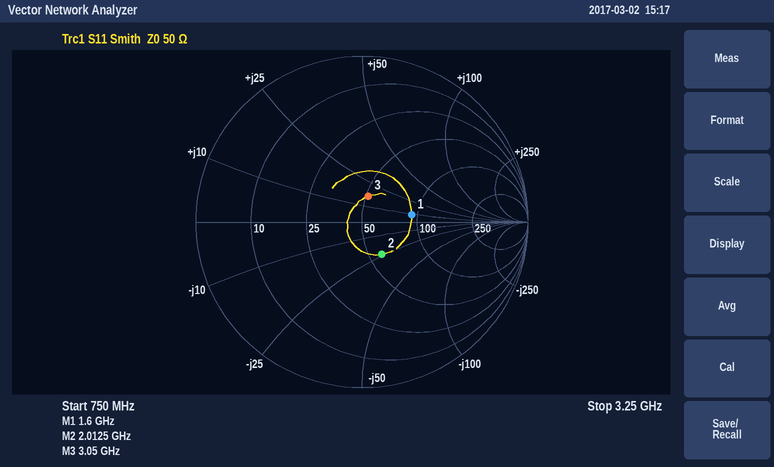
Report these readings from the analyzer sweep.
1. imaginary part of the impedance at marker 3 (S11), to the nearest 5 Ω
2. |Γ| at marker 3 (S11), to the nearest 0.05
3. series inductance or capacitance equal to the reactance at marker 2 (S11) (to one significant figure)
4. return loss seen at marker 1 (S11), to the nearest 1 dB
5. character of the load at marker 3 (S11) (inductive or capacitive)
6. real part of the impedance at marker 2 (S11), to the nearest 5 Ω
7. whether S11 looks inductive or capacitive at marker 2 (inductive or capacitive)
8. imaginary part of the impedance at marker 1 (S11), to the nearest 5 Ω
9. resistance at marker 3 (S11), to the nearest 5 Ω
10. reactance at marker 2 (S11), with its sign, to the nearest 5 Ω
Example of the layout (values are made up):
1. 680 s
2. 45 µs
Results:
1. +15 Ω
2. 0.15
3. 3 pF
4. 10 dB
5. inductive
6. 60 Ω
7. capacitive
8. +10 Ω
9. 50 Ω
10. -25 Ω
